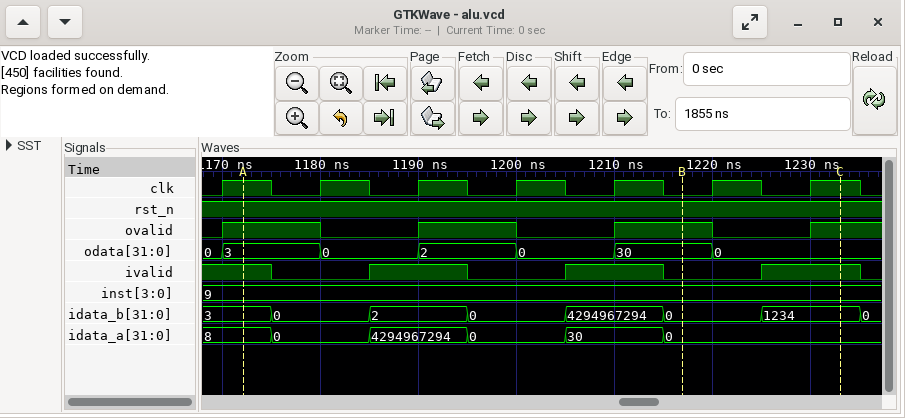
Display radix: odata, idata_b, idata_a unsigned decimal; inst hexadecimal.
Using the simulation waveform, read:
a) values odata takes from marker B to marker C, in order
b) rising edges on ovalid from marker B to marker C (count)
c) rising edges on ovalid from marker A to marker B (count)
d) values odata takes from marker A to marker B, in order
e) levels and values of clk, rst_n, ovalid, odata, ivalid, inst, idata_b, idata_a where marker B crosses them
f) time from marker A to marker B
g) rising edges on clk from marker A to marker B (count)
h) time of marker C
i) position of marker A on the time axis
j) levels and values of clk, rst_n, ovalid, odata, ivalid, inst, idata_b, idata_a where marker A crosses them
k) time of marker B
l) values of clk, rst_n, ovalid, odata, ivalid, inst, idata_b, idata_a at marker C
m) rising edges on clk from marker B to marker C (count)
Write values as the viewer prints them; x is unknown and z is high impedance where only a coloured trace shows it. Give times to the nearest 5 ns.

30, 0
1
2
3, 0, 2, 0, 30
clk=0, rst_n=1, ovalid=1, odata=30, ivalid=0, inst=9, idata_b=0, idata_a=0
45 ns
4
1235 ns
1170 ns
clk=1, rst_n=1, ovalid=1, odata=3, ivalid=1, inst=9, idata_b=3, idata_a=8
1215 ns
clk=1, rst_n=1, ovalid=1, odata=0, ivalid=1, inst=9, idata_b=1234, idata_a=0
2
